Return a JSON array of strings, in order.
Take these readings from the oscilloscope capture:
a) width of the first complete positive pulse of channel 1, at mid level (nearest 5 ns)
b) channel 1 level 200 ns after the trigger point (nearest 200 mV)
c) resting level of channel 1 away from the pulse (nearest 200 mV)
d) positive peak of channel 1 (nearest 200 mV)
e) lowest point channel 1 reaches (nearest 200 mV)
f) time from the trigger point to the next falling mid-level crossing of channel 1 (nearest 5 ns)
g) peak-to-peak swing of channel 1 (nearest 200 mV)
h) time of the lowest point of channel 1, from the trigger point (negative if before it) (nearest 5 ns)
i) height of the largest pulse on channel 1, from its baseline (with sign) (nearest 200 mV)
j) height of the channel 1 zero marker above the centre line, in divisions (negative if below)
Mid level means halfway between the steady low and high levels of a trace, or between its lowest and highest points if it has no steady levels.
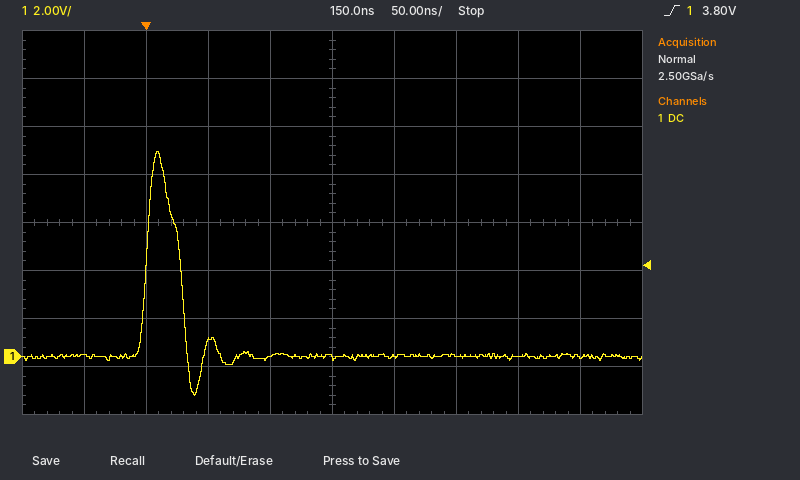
["30 ns", "0.0 V", "0.0 V", "8.6 V", "-1.6 V", "30 ns", "10.2 V", "+40 ns", "+8.6 V", "-2.8 div"]
